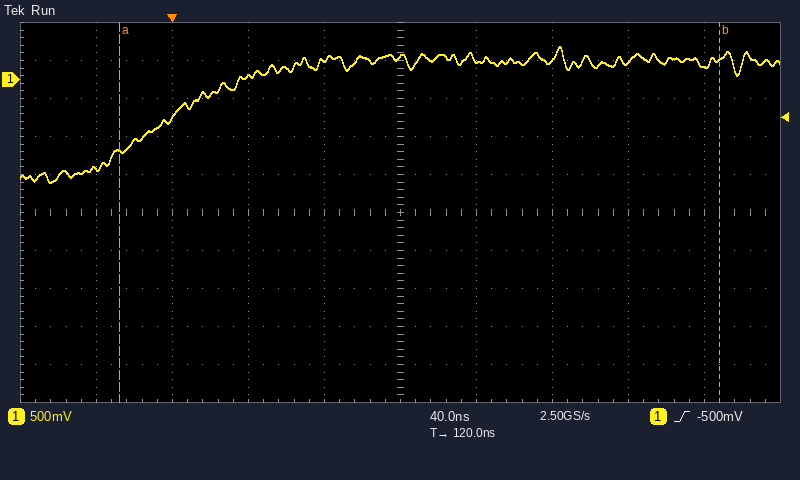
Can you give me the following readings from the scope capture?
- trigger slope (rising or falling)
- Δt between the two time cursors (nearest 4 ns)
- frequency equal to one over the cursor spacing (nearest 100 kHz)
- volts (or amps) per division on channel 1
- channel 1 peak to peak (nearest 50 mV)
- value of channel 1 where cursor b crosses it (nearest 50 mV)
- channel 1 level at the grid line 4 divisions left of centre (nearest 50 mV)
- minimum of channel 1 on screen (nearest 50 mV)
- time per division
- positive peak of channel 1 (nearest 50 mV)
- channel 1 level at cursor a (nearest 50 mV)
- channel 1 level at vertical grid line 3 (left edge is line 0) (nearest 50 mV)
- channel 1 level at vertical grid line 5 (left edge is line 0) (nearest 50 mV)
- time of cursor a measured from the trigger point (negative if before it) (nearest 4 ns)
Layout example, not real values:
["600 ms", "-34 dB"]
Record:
["rising", "316 ns", "3.2 MHz", "500 mV", "1.80 V", "250 mV", "-1.15 V", "-1.35 V", "40 ns", "450 mV", "-950 mV", "50 mV", "300 mV", "-28 ns"]
